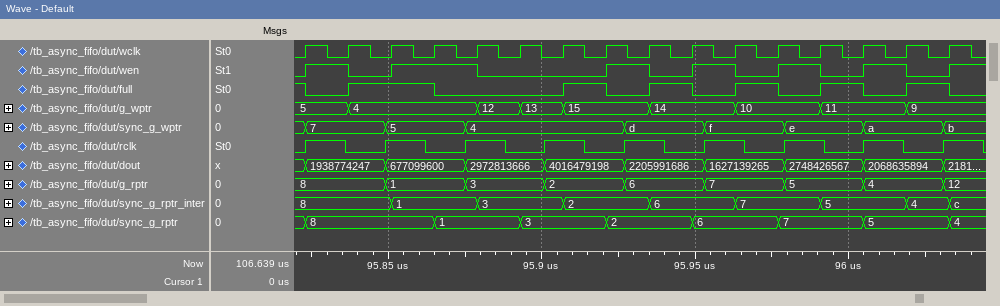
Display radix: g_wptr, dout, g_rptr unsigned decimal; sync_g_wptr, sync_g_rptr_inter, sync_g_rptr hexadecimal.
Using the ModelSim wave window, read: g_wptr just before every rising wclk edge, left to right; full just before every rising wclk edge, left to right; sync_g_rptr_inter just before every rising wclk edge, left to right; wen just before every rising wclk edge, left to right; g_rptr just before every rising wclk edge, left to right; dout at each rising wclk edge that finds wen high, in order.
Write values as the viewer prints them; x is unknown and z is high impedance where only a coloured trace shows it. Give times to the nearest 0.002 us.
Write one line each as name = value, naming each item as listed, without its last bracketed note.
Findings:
g_wptr just before every rising wclk edge, left to right = 5, 5, 4, 4, 4, 12, 13, 15, 15, 14, 14, 10, 10, 11, 11, 9
full just before every rising wclk edge, left to right = 1 0 1 1 0 0 0 1 0 1 0 1 0 1 0 1
sync_g_rptr_inter just before every rising wclk edge, left to right = 8, 8, 8, 1, 1, 3, 3, 2, 2, 6, 6, 7, 7, 5, 5, 4
wen just before every rising wclk edge, left to right = 0 1 0 1 1 0 0 0 1 0 1 0 1 0 1 0
g_rptr just before every rising wclk edge, left to right = 8, 8, 1, 1, 3, 3, 2, 2, 6, 6, 7, 7, 5, 5, 4, 12
dout at each rising wclk edge that finds wen high, in order = 1938774247, 677099600, 2972813666, 2205991686, 1627139265, 2748426567, 2068635894
